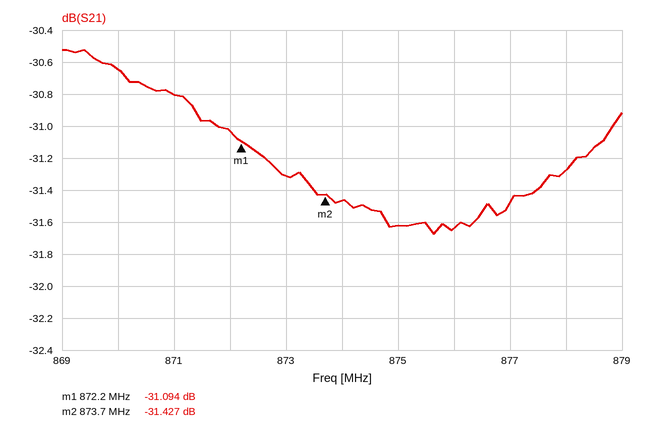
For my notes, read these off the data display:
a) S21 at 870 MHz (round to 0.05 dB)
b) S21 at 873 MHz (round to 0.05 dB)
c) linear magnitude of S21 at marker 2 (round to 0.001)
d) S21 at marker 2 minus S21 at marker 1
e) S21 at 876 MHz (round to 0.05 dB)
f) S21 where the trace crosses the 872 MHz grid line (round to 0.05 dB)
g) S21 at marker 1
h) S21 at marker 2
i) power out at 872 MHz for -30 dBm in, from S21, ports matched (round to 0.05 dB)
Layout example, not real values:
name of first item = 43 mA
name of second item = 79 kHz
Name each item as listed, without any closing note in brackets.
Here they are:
S21 at 870 MHz = -30.65 dB
S21 at 873 MHz = -31.30 dB
linear magnitude of S21 at marker 2 = 0.027
S21 at marker 2 minus S21 at marker 1 = -0.333 dB
S21 at 876 MHz = -31.65 dB
S21 where the trace crosses the 872 MHz grid line = -31.05 dB
S21 at marker 1 = -31.094 dB
S21 at marker 2 = -31.427 dB
power out at 872 MHz for -30 dBm in, from S21, ports matched = -61.05 dBm
